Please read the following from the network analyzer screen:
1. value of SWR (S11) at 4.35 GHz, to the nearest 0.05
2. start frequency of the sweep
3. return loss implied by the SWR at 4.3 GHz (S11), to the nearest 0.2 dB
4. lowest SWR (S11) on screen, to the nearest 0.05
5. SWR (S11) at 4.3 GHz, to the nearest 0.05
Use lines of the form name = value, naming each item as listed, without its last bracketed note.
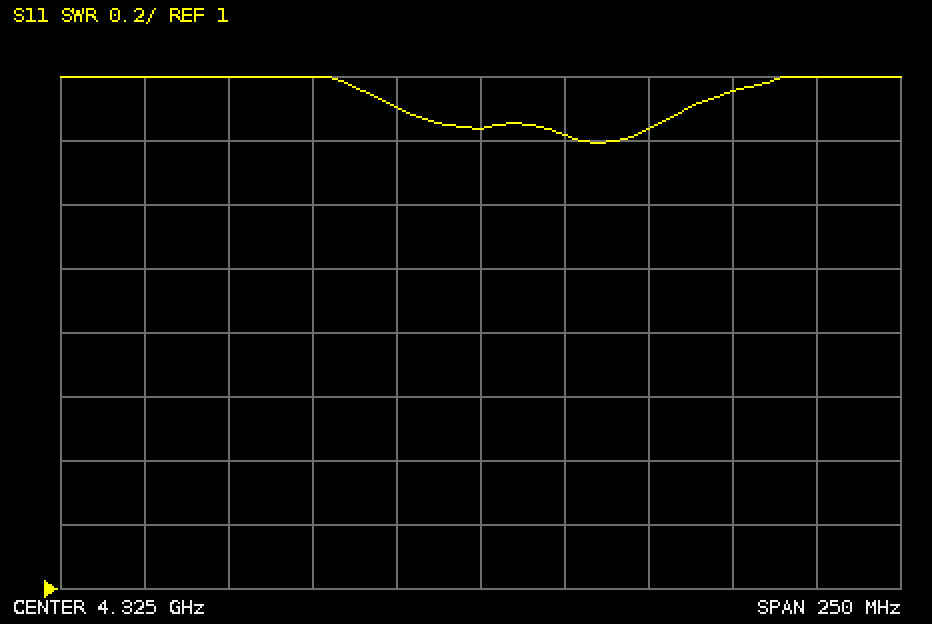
value of SWR (S11) at 4.35 GHz, to the nearest 0.05 = 2.40
start frequency of the sweep = 4.2 GHz
return loss implied by the SWR at 4.3 GHz (S11), to the nearest 0.2 dB = 7.4 dB
lowest SWR (S11) on screen, to the nearest 0.05 = 2.40
SWR (S11) at 4.3 GHz, to the nearest 0.05 = 2.50
